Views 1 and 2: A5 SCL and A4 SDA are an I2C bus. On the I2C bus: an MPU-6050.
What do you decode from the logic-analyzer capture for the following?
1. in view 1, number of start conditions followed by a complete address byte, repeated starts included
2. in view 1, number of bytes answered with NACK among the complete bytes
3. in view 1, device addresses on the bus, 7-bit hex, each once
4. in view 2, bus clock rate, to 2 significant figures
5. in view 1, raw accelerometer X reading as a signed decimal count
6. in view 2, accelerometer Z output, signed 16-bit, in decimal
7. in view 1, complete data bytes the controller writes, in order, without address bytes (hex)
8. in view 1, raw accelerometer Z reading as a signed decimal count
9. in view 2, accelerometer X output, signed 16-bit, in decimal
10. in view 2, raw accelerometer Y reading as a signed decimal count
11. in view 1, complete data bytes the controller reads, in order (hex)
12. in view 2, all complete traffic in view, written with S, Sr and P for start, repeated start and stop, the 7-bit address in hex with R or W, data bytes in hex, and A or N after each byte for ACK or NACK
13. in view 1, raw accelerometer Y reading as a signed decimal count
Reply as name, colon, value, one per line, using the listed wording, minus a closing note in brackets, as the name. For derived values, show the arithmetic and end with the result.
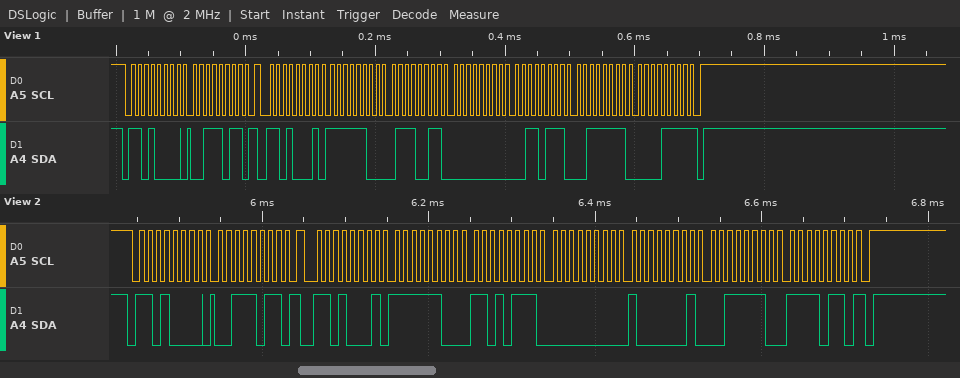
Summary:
in view 1, number of start conditions followed by a complete address byte, repeated starts included: 2
in view 1, number of bytes answered with NACK among the complete bytes: 1
in view 1, device addresses on the bus, 7-bit hex, each once: 0x68
in view 2, bus clock rate, to 2 significant figures: 100 kHz
in view 1, raw accelerometer X reading as a signed decimal count: 0xFC73 = -909
in view 2, accelerometer Z output, signed 16-bit, in decimal: 0x3EF6 = 16118
in view 1, complete data bytes the controller writes, in order, without address bytes: 3B
in view 1, raw accelerometer Z reading as a signed decimal count: 0x3F0F = 16143
in view 2, accelerometer X output, signed 16-bit, in decimal: 0xFCD7 = -809
in view 2, raw accelerometer Y reading as a signed decimal count: 0x0081 = 129
in view 1, complete data bytes the controller reads, in order: FC 73 00 37 3F 0F
in view 2, all complete traffic in view, written with S, Sr and P for start, repeated start and stop, the 7-bit address in hex with R or W, data bytes in hex, and A or N after each byte for ACK or NACK: S 68W A 3B A Sr 68R A FC A D7 A 00 A 81 A 3E A F6 N P
in view 1, raw accelerometer Y reading as a signed decimal count: 0x0037 = 55
